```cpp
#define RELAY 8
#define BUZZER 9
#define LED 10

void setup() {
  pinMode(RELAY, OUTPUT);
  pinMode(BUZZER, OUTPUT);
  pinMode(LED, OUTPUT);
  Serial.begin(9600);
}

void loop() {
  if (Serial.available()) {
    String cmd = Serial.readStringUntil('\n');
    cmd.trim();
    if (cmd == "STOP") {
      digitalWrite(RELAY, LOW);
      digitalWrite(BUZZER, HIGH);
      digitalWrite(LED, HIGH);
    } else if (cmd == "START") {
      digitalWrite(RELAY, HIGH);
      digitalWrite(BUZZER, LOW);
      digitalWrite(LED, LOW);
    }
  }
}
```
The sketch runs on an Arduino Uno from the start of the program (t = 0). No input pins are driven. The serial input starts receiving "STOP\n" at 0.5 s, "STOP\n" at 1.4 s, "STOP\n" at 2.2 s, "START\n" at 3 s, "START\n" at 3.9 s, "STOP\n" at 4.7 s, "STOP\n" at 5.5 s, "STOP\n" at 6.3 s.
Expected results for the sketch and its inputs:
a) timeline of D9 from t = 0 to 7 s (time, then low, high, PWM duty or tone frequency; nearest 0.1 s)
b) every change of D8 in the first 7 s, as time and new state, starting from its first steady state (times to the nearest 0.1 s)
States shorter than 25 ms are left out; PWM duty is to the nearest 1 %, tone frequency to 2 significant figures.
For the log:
0 s low; 0.5 s high; 3 s low; 4.7 s high
0 s low; 3 s high; 4.7 s low
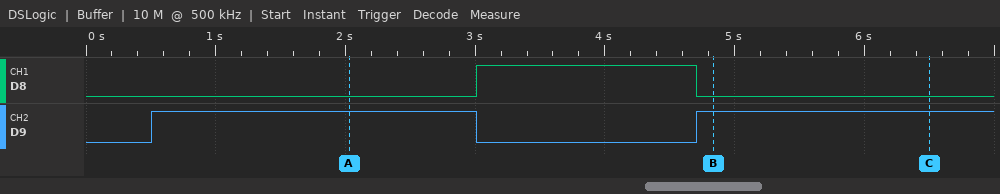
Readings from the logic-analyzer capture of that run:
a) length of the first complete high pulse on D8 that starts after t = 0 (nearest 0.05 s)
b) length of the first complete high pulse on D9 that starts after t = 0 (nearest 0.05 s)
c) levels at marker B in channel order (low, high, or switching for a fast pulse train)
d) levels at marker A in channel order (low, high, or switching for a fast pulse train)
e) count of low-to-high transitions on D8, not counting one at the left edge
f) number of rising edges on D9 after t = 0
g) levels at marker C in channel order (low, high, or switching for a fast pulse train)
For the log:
1.70 s
2.50 s
D8 low, D9 high
D8 low, D9 high
1
2
D8 low, D9 high
